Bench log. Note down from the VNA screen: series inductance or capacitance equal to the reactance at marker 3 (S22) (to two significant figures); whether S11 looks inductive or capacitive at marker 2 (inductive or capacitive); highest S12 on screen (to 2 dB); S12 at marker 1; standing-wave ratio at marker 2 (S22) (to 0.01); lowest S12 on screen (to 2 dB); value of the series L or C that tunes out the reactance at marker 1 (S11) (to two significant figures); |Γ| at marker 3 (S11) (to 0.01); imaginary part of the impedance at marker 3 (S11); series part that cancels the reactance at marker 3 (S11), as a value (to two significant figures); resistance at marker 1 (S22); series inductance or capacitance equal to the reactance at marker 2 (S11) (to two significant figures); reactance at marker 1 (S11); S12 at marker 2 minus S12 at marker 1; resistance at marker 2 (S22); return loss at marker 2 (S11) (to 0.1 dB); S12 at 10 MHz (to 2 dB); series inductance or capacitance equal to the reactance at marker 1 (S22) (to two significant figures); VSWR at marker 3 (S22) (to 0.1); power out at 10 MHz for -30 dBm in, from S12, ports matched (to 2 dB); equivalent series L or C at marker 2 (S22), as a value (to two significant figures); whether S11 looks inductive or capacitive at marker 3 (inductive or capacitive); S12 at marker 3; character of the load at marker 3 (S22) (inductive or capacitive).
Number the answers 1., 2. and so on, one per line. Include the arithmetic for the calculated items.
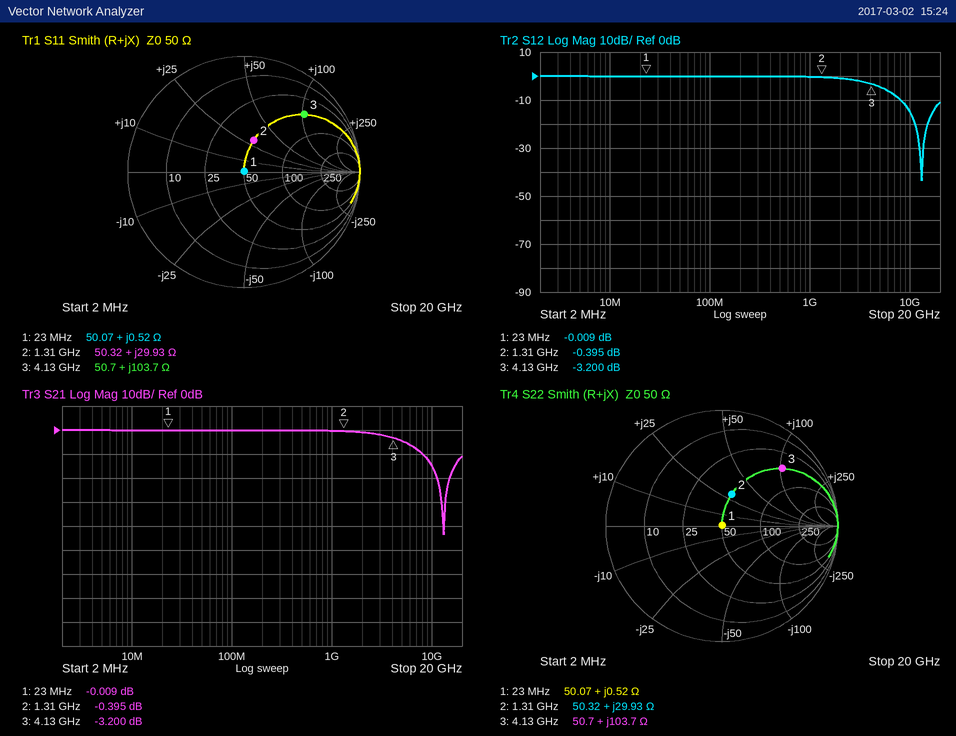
1. L = 103.7 Ω/(2π × 4.13 GHz) ≈ 4.0 nH
2. inductive
3. 0 dB
4. -0.009 dB
5. 1.80
6. -44 dB
7. C = 1/(2π × 23 MHz × 0.52 Ω) ≈ 13 nF
8. 0.72
9. +103.7 Ω
10. C = 1/(2π × 4.13 GHz × 103.7 Ω) ≈ 372 fF, so 370 fF to two significant figures
11. 50.07 Ω
12. L = 29.93 Ω/(2π × 1.31 GHz) ≈ 3.6 nH
13. +0.52 Ω
14. -0.395 − (-0.009) = -0.386 dB
15. 50.32 Ω
16. 10.9 dB
17. 0 dB
18. L = 0.52 Ω/(2π × 23 MHz) ≈ 3.6 nH
19. 6.1
20. -30 dBm + (0 dB) = -30 dBm
21. L = 29.93 Ω/(2π × 1.31 GHz) ≈ 3.6 nH
22. inductive
23. -3.200 dB
24. inductive
